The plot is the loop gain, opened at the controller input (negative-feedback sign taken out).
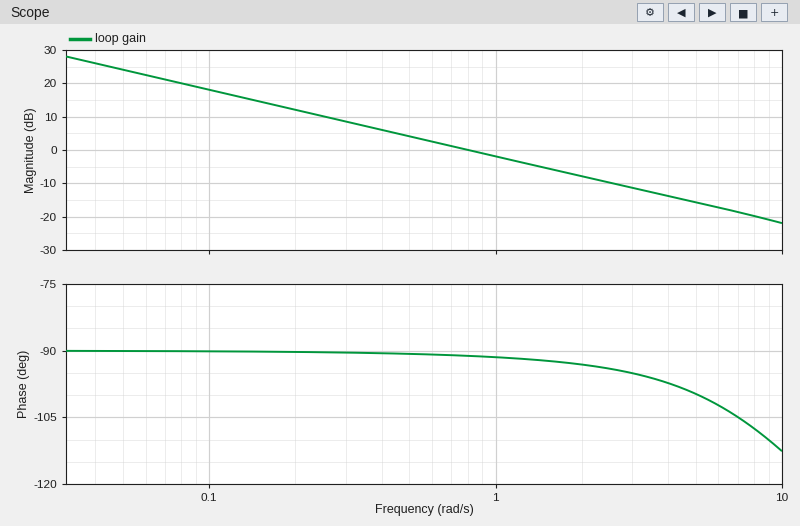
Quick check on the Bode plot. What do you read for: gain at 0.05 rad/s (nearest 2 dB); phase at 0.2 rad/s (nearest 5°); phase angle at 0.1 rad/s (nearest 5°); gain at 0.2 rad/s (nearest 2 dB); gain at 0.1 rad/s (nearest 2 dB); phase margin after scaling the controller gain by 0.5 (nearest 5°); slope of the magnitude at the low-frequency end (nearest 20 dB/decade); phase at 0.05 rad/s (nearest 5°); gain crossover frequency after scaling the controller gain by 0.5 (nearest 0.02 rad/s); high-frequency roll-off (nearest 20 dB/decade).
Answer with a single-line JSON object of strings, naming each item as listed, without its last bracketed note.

{"gain at 0.05 rad/s": "24 dB", "phase at 0.2 rad/s": "-90°", "phase angle at 0.1 rad/s": "-90°", "gain at 0.2 rad/s": "12 dB", "gain at 0.1 rad/s": "18 dB", "phase margin after scaling the controller gain by 0.5": "90°", "slope of the magnitude at the low-frequency end": "-20 dB/decade", "phase at 0.05 rad/s": "-90°", "gain crossover frequency after scaling the controller gain by 0.5": "0.40 rad/s", "high-frequency roll-off": "-20 dB/decade"}
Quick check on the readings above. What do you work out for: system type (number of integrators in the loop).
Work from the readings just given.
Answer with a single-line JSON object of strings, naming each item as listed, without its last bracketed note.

{"system type": "1"}
